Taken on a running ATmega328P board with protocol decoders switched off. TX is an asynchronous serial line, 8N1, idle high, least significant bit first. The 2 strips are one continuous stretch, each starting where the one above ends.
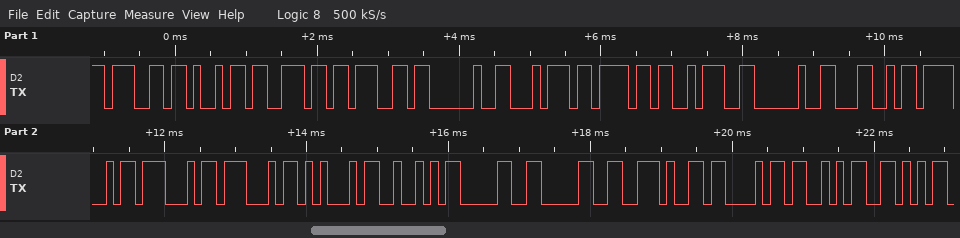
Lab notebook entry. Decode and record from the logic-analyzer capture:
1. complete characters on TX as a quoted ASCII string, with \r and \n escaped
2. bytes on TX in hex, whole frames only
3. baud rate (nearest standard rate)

"ging to: LOGGER00.CSV"
67 69 6E 67 20 74 6F 3A 20 4C 4F 47 47 45 52 30 30 2E 43 53 56
9600 baud
